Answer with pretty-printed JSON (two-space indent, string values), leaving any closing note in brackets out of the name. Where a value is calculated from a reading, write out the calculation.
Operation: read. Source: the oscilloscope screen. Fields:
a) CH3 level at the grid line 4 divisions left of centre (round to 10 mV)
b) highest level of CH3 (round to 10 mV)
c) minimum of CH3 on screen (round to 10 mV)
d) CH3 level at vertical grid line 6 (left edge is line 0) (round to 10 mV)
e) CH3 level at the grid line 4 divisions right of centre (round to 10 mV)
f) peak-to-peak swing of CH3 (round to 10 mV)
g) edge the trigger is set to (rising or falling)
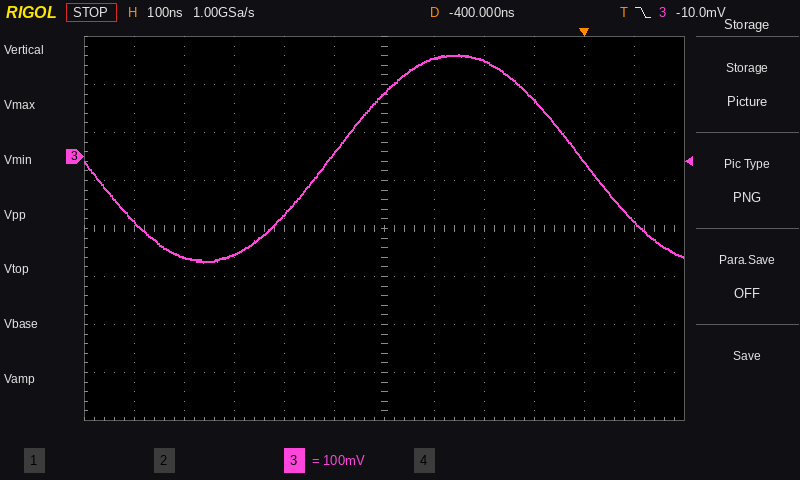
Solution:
{
  "CH3 level at the grid line 4 divisions left of centre": "-210 mV",
  "highest level of CH3": "210 mV",
  "minimum of CH3 on screen": "-220 mV",
  "CH3 level at vertical grid line 6 (left edge is line 0)": "130 mV",
  "CH3 level at the grid line 4 divisions right of centre": "-10 mV",
  "peak-to-peak swing of CH3": "210 mV − (-220 mV) = 430 mV",
  "edge the trigger is set to": "falling"
}
